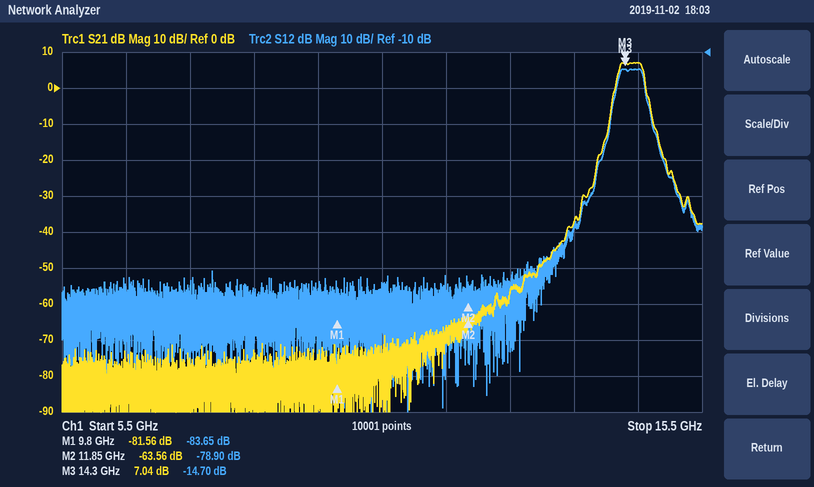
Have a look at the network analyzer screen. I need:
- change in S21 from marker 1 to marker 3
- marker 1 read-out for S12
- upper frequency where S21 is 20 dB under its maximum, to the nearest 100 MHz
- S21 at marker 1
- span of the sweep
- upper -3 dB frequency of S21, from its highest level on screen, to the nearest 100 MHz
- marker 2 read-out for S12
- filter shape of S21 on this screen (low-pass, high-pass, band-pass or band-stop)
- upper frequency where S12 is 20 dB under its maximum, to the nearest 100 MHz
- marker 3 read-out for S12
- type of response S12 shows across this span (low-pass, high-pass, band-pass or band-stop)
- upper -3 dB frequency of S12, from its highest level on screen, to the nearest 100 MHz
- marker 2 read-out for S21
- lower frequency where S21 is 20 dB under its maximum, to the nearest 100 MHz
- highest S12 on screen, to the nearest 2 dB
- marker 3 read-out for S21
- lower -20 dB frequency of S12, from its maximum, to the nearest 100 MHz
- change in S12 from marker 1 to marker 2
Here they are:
88.60 dB
-83.65 dB
14.8 GHz
-81.56 dB
10 GHz
14.6 GHz
-78.90 dB
band-pass
14.8 GHz
-14.70 dB
band-pass
14.6 GHz
-63.56 dB
14.0 GHz
-14 dB
7.04 dB
14.0 GHz
4.75 dB
